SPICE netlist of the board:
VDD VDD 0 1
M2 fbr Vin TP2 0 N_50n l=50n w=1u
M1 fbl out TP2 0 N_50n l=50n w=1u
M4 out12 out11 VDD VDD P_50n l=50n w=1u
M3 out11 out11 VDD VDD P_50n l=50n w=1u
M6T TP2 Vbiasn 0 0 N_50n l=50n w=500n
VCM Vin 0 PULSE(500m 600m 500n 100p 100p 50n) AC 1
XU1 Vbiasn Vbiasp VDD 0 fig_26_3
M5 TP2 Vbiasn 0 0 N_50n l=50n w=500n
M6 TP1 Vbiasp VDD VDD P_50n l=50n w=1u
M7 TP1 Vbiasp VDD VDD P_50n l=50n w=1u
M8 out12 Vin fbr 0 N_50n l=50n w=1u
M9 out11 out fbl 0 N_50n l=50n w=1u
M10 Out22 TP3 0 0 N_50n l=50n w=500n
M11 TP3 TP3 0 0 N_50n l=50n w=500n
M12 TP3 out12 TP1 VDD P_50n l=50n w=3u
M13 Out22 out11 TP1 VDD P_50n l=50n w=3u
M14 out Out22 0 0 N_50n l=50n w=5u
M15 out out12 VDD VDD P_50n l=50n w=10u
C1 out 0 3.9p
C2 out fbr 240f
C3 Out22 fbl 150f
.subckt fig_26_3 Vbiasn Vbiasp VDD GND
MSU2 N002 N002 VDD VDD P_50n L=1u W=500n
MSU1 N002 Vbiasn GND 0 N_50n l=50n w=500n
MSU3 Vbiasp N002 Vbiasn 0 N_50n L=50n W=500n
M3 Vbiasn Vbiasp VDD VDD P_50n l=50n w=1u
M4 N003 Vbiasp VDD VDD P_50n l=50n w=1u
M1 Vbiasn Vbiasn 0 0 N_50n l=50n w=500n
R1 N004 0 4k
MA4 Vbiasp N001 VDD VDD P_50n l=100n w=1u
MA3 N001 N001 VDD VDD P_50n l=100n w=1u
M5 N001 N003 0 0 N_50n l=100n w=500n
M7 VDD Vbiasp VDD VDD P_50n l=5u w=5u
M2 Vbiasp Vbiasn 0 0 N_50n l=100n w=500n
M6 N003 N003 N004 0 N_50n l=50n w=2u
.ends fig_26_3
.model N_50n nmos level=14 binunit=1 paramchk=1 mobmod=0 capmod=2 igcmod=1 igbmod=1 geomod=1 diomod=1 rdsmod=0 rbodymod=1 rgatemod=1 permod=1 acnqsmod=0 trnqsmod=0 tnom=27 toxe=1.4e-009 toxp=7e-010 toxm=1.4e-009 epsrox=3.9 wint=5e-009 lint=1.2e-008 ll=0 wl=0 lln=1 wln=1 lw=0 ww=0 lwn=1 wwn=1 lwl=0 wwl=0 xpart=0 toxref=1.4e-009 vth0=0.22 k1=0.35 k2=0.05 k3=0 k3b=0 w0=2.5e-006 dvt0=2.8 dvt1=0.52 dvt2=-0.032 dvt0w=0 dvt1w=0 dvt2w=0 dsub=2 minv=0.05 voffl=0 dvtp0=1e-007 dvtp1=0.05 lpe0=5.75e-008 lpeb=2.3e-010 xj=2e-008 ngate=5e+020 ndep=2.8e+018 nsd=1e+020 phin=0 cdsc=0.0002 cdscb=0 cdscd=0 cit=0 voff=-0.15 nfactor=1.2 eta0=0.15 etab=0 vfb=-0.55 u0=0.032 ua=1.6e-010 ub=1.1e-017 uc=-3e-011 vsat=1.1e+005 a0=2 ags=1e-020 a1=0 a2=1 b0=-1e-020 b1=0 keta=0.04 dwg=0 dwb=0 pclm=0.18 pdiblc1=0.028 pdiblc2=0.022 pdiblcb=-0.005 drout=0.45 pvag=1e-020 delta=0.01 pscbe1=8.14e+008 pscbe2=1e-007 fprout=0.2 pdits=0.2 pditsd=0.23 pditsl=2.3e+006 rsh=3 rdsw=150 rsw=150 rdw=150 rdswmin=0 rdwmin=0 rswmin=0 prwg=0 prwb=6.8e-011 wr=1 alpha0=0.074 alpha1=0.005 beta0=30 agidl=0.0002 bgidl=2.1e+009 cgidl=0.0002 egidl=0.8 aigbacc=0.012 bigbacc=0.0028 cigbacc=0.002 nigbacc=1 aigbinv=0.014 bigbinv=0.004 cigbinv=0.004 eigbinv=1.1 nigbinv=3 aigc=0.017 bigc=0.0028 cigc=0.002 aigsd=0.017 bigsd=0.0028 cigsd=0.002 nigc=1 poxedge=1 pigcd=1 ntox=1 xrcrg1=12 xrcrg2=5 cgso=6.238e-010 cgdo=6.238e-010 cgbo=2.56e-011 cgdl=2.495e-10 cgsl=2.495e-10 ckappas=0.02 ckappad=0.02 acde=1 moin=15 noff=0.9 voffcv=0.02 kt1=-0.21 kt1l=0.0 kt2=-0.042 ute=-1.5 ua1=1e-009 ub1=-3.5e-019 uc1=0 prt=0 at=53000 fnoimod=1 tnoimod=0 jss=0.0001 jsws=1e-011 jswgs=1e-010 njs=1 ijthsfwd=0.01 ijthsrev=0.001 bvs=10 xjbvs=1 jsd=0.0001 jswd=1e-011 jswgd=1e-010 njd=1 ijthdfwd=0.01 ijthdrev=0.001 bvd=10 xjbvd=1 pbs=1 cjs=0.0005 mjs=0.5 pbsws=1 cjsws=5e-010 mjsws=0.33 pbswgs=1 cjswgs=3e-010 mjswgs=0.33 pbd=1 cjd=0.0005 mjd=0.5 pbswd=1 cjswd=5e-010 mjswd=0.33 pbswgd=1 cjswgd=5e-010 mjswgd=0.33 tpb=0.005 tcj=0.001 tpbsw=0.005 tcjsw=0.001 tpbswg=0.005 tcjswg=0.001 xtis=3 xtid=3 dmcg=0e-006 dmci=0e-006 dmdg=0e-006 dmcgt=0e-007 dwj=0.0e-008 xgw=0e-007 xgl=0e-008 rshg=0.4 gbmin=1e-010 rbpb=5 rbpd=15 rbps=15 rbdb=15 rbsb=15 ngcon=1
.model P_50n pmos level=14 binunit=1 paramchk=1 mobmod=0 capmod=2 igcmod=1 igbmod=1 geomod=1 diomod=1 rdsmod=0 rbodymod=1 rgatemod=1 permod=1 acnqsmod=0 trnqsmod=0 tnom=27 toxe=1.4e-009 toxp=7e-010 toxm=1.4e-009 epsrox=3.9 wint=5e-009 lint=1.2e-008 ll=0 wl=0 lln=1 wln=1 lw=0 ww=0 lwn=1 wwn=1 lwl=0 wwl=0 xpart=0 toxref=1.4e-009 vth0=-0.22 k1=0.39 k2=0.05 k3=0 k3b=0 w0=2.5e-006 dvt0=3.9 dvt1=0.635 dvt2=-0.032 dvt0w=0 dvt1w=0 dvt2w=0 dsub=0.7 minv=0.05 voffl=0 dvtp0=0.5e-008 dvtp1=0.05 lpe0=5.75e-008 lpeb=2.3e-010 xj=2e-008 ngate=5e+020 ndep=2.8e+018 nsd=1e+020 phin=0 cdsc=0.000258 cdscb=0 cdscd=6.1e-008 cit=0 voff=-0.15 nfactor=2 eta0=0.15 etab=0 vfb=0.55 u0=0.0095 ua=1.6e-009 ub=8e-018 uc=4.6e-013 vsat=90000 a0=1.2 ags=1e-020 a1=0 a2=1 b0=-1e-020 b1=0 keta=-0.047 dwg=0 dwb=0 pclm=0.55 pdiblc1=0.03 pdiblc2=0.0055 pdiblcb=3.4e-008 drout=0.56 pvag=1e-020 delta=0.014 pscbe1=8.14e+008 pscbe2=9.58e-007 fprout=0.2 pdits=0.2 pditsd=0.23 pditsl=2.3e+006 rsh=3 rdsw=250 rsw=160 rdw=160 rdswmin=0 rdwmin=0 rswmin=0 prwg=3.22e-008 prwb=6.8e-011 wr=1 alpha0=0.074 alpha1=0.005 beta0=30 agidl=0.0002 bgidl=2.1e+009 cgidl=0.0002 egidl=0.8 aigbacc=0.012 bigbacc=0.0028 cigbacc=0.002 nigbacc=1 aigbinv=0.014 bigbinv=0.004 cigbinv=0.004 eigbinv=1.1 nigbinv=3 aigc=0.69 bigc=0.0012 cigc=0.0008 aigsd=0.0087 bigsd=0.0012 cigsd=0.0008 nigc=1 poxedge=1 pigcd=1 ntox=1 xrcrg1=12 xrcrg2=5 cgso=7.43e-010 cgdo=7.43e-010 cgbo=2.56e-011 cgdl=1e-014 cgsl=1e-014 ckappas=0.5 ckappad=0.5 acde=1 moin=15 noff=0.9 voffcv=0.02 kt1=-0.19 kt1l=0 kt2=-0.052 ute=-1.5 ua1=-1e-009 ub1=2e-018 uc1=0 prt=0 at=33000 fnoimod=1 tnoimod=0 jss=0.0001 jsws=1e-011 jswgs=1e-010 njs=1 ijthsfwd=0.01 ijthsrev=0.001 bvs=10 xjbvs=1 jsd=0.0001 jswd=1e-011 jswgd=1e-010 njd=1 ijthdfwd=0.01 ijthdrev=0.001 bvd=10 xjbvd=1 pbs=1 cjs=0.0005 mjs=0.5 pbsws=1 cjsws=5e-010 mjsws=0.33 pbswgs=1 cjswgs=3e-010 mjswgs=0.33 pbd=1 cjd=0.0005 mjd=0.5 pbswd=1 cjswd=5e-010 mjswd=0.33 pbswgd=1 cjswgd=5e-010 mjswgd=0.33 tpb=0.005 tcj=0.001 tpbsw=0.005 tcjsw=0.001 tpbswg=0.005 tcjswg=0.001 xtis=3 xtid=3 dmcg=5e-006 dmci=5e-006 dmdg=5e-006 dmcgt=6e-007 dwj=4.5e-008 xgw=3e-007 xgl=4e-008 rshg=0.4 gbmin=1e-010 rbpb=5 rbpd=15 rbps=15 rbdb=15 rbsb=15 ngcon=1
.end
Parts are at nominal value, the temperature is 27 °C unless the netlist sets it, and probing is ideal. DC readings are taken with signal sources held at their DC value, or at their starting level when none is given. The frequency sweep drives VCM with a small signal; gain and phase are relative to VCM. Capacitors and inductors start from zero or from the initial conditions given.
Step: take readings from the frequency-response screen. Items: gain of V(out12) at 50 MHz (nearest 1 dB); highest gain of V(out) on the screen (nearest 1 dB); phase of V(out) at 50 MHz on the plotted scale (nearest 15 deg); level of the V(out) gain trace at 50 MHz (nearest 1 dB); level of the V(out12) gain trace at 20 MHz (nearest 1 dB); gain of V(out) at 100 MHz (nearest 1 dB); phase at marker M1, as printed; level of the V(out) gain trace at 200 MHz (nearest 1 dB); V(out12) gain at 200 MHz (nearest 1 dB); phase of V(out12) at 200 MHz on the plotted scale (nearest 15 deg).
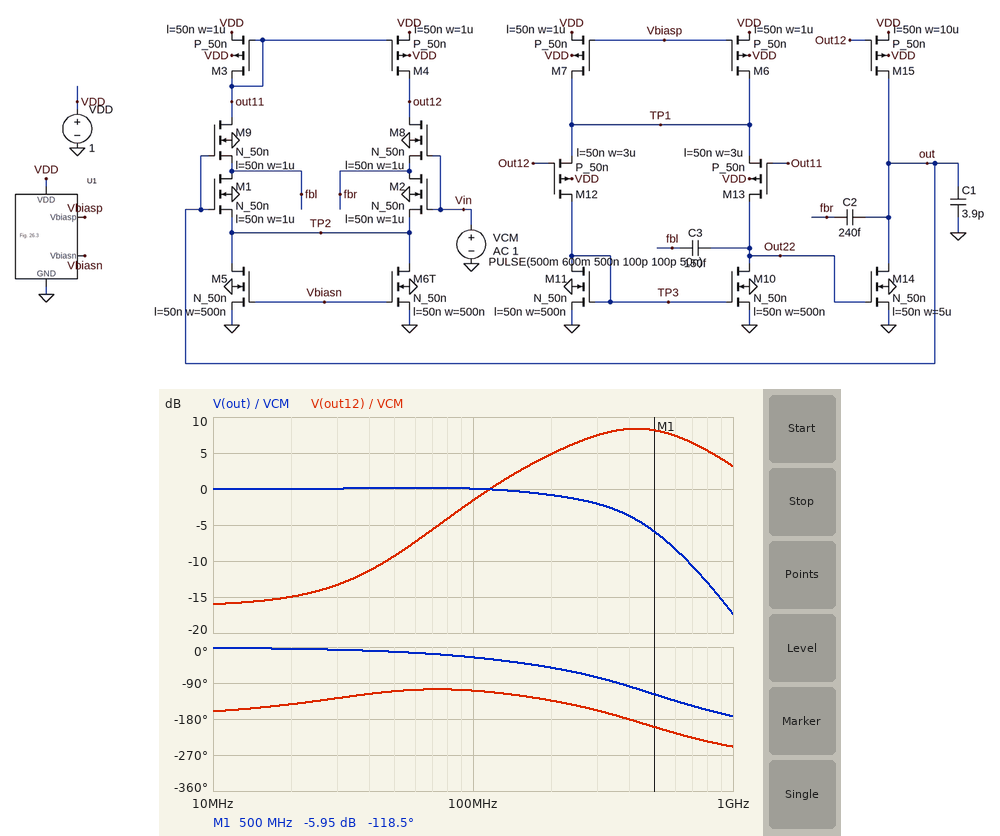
-9 dB
0 dB
-15 deg
0 dB
-15 dB
0 dB
-118.5 deg
-1 dB
5 dB
-135 deg
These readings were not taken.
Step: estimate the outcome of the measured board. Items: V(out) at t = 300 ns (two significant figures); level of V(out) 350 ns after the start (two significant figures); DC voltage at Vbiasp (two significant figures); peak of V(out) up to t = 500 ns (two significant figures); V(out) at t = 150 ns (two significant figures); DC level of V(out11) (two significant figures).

500 mV
500 mV
590 mV
630 mV
500 mV
600 mV
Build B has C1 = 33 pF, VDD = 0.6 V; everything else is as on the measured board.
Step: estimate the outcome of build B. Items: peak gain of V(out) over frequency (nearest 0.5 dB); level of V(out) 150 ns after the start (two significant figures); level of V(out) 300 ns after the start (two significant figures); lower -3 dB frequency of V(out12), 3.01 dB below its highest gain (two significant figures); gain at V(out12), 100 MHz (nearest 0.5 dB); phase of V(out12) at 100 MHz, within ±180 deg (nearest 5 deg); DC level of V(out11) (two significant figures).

4.5 dB
400 mV
480 mV
34 MHz
6.0 dB
170 deg
210 mV
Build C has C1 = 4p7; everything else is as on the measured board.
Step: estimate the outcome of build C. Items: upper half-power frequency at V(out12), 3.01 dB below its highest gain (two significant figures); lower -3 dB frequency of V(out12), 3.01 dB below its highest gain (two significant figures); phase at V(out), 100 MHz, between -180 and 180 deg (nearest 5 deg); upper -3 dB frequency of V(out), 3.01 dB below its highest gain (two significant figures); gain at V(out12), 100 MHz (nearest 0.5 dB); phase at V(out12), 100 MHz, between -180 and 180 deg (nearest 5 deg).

750 MHz
180 MHz
-30 deg
290 MHz
0 dB
-105 deg
